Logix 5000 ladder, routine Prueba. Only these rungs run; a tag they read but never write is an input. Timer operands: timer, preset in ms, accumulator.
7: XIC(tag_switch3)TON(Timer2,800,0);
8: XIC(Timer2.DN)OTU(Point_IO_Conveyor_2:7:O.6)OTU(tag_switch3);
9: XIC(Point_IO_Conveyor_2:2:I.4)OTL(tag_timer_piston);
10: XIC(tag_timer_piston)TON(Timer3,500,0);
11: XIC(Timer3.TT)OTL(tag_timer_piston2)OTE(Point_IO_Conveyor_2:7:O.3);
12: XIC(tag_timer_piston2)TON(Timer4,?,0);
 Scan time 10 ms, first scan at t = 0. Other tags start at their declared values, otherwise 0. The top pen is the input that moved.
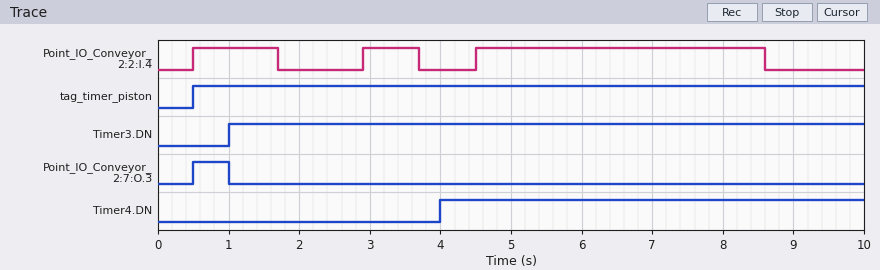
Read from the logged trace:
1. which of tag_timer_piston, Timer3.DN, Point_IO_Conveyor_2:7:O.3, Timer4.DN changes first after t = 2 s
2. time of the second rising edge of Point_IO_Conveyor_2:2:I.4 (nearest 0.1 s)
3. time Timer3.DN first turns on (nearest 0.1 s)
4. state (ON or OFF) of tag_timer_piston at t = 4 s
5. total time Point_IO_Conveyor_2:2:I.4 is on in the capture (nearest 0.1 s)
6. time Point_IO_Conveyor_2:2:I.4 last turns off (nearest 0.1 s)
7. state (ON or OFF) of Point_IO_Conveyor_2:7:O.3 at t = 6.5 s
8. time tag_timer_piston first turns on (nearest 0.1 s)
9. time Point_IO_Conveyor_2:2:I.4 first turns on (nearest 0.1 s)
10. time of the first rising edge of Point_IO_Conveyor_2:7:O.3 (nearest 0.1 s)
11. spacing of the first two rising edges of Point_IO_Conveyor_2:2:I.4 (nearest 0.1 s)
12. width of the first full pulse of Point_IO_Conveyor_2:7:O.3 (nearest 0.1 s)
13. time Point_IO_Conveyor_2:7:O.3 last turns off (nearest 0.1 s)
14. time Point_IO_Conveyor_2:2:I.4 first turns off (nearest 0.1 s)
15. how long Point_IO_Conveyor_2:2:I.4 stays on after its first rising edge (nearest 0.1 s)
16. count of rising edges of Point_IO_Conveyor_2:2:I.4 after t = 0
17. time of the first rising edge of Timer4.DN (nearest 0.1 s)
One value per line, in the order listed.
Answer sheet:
Timer4.DN
2.9 s
1.0 s
ON
6.1 s
8.6 s
OFF
0.5 s
0.5 s
0.5 s
2.4 s
0.5 s
1.0 s
1.7 s
1.2 s
3
4.0 s
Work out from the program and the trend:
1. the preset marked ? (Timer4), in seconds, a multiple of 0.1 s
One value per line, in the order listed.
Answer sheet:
3.5 s
